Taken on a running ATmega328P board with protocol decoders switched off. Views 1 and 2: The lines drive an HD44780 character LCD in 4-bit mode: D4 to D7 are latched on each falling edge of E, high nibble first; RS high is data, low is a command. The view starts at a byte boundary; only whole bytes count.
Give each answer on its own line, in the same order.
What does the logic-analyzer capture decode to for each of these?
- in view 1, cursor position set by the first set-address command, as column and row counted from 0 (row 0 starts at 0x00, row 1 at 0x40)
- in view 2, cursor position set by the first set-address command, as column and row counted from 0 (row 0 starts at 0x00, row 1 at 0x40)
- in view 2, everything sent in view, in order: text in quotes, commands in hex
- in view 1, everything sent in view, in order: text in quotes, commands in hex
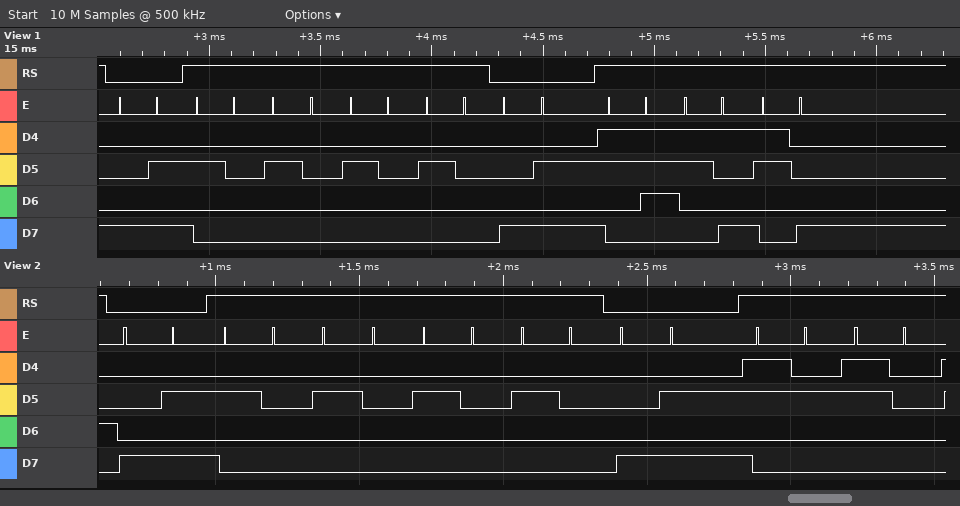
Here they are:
column 10, row 0
column 10, row 0
0x8A "    " 0x8A "20"
0x8A "    " 0x8A "798"
